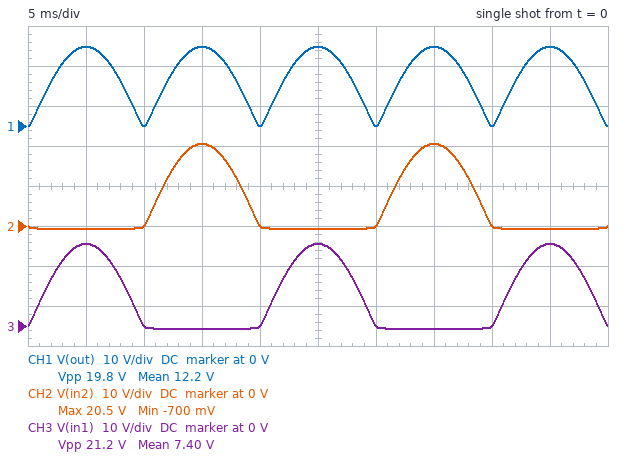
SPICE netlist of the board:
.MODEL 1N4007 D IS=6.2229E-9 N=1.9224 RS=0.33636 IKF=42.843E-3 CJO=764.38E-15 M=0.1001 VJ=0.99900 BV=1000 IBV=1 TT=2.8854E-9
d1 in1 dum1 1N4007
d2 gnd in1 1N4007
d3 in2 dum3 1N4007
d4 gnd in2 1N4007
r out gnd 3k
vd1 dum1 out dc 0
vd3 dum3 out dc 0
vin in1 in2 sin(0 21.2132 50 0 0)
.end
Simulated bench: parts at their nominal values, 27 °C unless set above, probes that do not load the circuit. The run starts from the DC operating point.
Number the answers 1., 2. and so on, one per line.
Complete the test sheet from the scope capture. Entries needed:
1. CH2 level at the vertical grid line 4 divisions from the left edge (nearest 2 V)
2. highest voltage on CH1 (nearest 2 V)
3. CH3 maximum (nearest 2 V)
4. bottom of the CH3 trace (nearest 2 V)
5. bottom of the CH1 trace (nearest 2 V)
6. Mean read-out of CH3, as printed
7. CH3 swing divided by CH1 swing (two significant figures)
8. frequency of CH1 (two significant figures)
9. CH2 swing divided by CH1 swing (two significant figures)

1. 0 V
2. 20 V
3. 20 V
4. 0 V
5. 0 V
6. 7.40 V
7. 1.1
8. 100 Hz
9. 1.1
